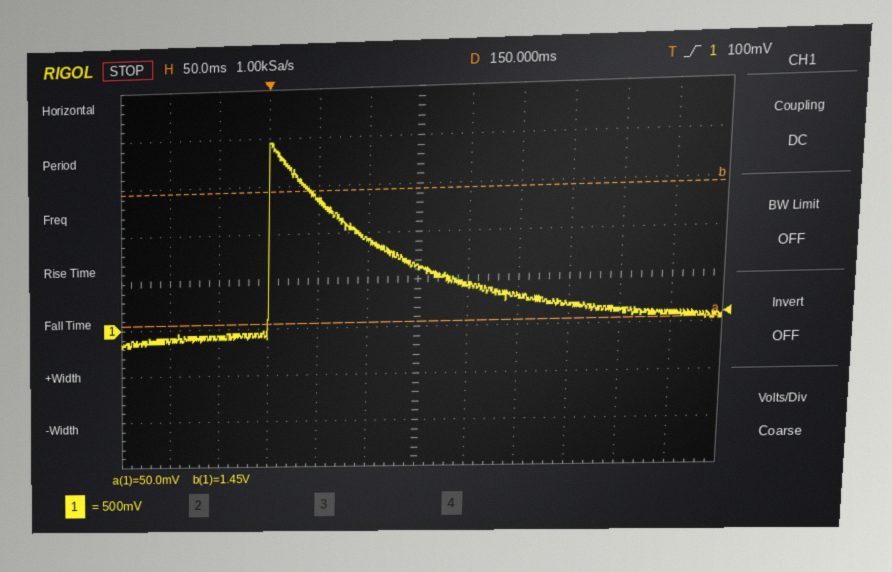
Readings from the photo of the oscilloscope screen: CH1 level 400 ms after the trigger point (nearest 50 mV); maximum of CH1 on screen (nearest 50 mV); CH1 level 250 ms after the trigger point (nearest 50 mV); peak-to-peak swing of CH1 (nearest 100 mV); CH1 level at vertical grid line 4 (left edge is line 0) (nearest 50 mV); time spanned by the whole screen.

100 mV
1.95 V
300 mV
2.10 V
1.35 V
600 ms
